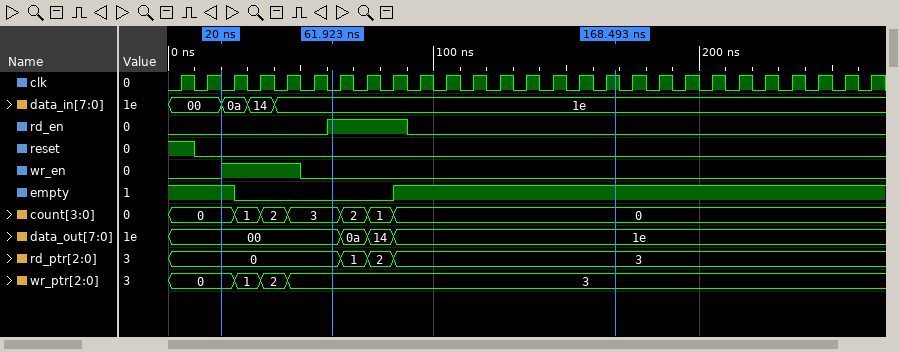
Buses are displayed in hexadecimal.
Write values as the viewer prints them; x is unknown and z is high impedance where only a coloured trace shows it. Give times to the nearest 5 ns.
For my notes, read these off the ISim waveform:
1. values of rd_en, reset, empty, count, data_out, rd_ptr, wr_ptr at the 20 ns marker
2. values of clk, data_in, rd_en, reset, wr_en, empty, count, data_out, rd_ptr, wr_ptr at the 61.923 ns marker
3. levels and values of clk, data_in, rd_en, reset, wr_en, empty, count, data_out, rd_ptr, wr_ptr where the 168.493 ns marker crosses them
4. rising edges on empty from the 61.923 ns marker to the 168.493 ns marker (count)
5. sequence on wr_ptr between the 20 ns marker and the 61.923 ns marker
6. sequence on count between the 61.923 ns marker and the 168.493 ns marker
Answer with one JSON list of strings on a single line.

["rd_en=0, reset=0, empty=1, count=0, data_out=00, rd_ptr=0, wr_ptr=0", "clk=0, data_in=1e, rd_en=1, reset=0, wr_en=0, empty=0, count=3, data_out=00, rd_ptr=0, wr_ptr=3", "clk=1, data_in=1e, rd_en=0, reset=0, wr_en=0, empty=1, count=0, data_out=1e, rd_ptr=3, wr_ptr=3", "1", "0, 1, 2, 3", "3, 2, 1, 0"]
